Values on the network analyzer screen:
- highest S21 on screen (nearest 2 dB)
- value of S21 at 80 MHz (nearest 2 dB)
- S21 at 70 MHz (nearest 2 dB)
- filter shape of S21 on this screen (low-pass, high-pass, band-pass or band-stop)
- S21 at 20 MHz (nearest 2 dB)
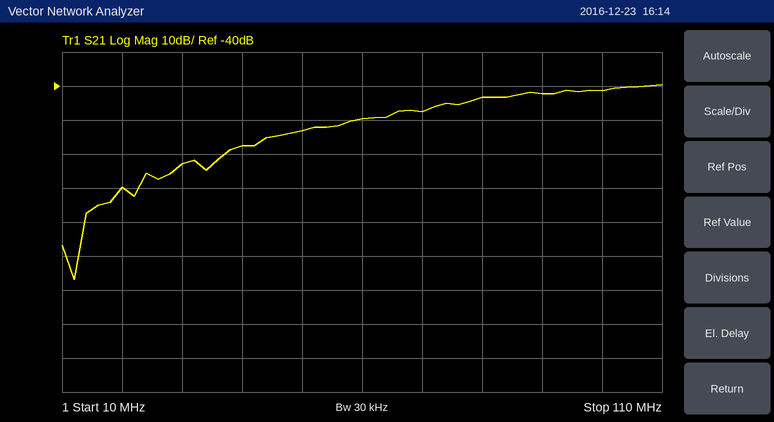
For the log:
-40 dB
-44 dB
-48 dB
high-pass
-70 dB
